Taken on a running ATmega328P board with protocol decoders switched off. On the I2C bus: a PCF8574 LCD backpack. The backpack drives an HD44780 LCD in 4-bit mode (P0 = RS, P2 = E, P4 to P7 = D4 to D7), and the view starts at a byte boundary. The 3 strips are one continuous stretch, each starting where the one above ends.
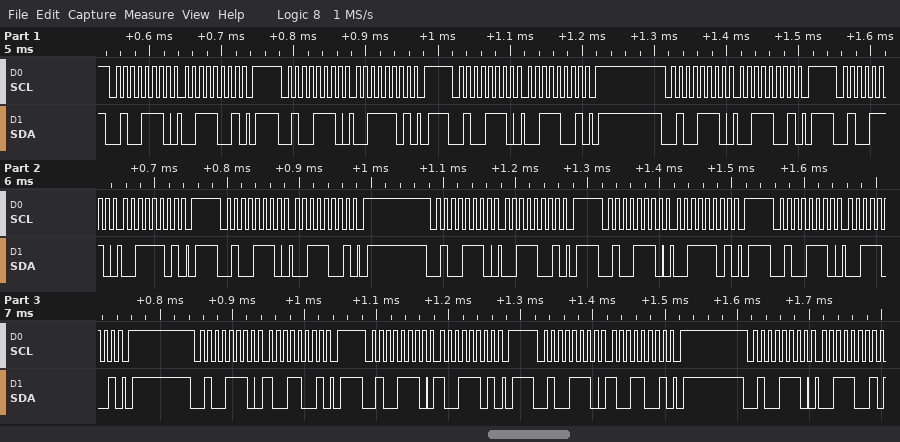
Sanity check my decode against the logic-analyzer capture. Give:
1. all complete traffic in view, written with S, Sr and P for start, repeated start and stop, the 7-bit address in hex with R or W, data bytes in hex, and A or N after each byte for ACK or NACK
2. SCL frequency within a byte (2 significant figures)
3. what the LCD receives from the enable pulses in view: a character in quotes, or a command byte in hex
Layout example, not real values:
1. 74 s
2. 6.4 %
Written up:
1. S 27W A 39 A P S 27W A 3D A P S 27W A 39 A P S 27W A 39 A P S 27W A 3D A P S 27W A 39 A P S 27W A 39 A P S 27W A 3D A P S 27W A 39 A P S 27W A 99 A P S 27W A 9D A P S 27W A 99 A P S 27W A 39 A
2. 100 kHz
3. '3' '9'
